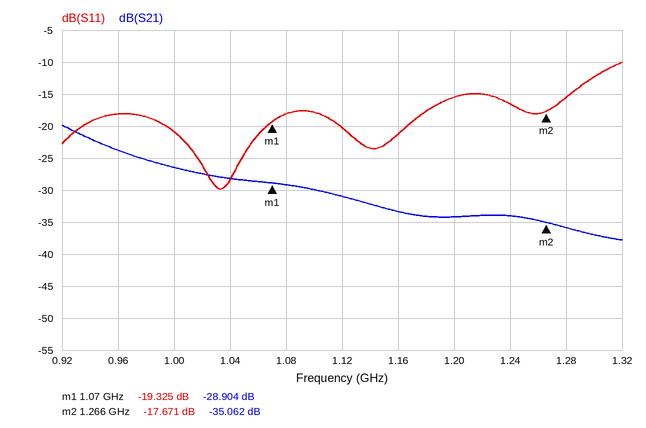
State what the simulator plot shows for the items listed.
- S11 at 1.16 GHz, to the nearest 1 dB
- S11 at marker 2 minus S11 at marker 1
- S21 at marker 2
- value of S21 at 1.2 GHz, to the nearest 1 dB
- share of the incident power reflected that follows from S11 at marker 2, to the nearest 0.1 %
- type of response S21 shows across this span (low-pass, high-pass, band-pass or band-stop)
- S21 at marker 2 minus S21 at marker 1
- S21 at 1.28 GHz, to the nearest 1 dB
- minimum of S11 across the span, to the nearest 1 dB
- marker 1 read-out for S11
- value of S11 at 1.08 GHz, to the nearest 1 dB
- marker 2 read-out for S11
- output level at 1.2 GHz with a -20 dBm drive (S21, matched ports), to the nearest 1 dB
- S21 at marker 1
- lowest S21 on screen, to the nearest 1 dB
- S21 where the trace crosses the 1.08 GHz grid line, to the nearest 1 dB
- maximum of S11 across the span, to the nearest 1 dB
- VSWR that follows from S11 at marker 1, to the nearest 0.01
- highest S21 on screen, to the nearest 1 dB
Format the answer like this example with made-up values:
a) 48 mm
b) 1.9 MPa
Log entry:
a) -21 dB
b) 1.654 dB
c) -35.062 dB
d) -34 dB
e) 1.7 %
f) low-pass
g) -6.158 dB
h) -36 dB
i) -30 dB
j) -19.325 dB
k) -18 dB
l) -17.671 dB
m) -54 dBm
n) -28.904 dB
o) -38 dB
p) -29 dB
q) -10 dB
r) 1.24
s) -20 dB
